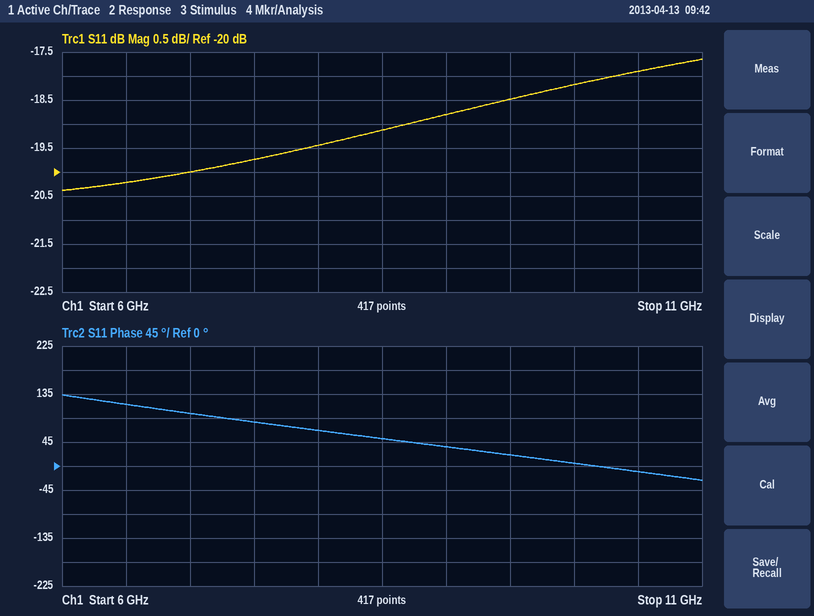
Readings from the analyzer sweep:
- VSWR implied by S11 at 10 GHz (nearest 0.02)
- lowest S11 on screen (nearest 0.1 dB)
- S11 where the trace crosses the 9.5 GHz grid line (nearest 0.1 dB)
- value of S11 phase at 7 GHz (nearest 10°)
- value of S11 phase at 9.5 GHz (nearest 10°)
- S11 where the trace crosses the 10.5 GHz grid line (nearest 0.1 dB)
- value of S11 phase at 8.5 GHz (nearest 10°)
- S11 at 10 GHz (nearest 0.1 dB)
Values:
1.28
-20.4 dB
-18.5 dB
100°
20°
-17.9 dB
50°
-18.2 dB
